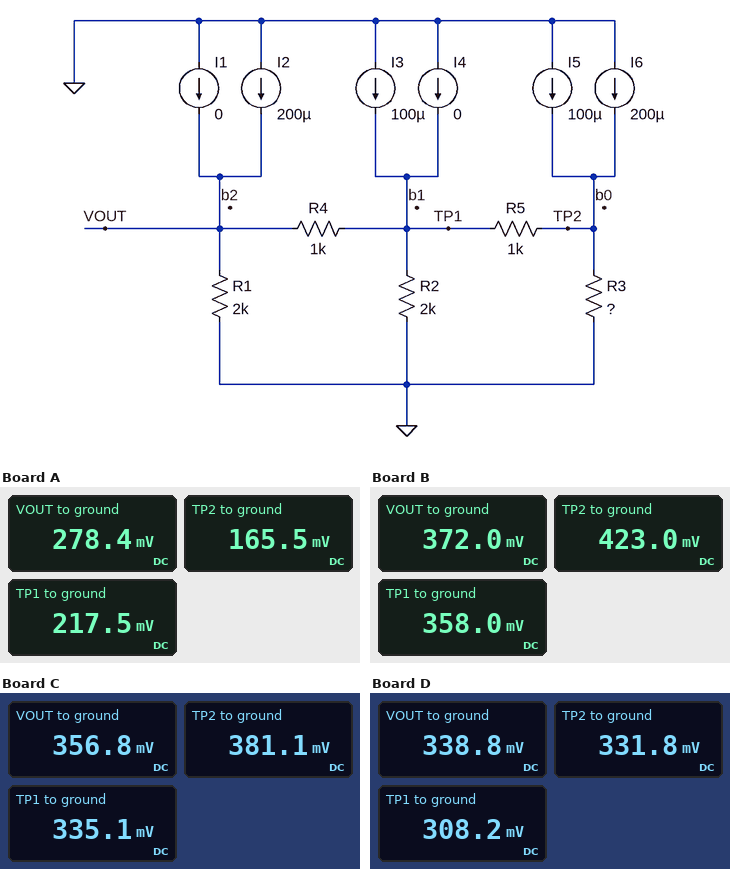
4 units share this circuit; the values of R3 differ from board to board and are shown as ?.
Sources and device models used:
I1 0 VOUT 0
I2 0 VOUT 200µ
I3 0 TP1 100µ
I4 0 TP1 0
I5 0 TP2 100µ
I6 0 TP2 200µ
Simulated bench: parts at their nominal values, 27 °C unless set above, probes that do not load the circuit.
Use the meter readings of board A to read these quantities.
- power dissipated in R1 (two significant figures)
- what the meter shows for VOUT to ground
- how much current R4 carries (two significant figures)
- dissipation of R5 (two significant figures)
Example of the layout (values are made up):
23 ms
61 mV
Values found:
39 µW
278.4 mV
61 µA
2.7 µW
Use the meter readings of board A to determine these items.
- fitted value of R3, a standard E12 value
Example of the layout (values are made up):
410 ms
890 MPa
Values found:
470 Ω
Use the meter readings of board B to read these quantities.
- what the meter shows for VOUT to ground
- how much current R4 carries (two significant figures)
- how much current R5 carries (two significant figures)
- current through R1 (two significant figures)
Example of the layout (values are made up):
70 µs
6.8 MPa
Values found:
372.0 mV
14 µA
65 µA
190 µA
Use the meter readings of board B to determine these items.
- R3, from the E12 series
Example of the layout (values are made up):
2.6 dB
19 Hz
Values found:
1.8 kΩ
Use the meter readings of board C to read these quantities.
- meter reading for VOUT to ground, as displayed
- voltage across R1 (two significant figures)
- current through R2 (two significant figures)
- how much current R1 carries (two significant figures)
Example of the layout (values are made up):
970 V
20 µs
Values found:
356.8 mV
360 mV
170 µA
180 µA
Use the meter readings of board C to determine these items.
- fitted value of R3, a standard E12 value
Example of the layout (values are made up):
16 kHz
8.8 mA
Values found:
1.5 kΩ
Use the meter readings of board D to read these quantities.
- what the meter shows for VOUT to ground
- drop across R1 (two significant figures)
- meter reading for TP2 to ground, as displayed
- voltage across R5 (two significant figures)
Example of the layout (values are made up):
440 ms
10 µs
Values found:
338.8 mV
340 mV
331.8 mV
24 mV
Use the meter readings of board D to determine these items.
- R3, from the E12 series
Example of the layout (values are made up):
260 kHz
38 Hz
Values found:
1.2 kΩ
